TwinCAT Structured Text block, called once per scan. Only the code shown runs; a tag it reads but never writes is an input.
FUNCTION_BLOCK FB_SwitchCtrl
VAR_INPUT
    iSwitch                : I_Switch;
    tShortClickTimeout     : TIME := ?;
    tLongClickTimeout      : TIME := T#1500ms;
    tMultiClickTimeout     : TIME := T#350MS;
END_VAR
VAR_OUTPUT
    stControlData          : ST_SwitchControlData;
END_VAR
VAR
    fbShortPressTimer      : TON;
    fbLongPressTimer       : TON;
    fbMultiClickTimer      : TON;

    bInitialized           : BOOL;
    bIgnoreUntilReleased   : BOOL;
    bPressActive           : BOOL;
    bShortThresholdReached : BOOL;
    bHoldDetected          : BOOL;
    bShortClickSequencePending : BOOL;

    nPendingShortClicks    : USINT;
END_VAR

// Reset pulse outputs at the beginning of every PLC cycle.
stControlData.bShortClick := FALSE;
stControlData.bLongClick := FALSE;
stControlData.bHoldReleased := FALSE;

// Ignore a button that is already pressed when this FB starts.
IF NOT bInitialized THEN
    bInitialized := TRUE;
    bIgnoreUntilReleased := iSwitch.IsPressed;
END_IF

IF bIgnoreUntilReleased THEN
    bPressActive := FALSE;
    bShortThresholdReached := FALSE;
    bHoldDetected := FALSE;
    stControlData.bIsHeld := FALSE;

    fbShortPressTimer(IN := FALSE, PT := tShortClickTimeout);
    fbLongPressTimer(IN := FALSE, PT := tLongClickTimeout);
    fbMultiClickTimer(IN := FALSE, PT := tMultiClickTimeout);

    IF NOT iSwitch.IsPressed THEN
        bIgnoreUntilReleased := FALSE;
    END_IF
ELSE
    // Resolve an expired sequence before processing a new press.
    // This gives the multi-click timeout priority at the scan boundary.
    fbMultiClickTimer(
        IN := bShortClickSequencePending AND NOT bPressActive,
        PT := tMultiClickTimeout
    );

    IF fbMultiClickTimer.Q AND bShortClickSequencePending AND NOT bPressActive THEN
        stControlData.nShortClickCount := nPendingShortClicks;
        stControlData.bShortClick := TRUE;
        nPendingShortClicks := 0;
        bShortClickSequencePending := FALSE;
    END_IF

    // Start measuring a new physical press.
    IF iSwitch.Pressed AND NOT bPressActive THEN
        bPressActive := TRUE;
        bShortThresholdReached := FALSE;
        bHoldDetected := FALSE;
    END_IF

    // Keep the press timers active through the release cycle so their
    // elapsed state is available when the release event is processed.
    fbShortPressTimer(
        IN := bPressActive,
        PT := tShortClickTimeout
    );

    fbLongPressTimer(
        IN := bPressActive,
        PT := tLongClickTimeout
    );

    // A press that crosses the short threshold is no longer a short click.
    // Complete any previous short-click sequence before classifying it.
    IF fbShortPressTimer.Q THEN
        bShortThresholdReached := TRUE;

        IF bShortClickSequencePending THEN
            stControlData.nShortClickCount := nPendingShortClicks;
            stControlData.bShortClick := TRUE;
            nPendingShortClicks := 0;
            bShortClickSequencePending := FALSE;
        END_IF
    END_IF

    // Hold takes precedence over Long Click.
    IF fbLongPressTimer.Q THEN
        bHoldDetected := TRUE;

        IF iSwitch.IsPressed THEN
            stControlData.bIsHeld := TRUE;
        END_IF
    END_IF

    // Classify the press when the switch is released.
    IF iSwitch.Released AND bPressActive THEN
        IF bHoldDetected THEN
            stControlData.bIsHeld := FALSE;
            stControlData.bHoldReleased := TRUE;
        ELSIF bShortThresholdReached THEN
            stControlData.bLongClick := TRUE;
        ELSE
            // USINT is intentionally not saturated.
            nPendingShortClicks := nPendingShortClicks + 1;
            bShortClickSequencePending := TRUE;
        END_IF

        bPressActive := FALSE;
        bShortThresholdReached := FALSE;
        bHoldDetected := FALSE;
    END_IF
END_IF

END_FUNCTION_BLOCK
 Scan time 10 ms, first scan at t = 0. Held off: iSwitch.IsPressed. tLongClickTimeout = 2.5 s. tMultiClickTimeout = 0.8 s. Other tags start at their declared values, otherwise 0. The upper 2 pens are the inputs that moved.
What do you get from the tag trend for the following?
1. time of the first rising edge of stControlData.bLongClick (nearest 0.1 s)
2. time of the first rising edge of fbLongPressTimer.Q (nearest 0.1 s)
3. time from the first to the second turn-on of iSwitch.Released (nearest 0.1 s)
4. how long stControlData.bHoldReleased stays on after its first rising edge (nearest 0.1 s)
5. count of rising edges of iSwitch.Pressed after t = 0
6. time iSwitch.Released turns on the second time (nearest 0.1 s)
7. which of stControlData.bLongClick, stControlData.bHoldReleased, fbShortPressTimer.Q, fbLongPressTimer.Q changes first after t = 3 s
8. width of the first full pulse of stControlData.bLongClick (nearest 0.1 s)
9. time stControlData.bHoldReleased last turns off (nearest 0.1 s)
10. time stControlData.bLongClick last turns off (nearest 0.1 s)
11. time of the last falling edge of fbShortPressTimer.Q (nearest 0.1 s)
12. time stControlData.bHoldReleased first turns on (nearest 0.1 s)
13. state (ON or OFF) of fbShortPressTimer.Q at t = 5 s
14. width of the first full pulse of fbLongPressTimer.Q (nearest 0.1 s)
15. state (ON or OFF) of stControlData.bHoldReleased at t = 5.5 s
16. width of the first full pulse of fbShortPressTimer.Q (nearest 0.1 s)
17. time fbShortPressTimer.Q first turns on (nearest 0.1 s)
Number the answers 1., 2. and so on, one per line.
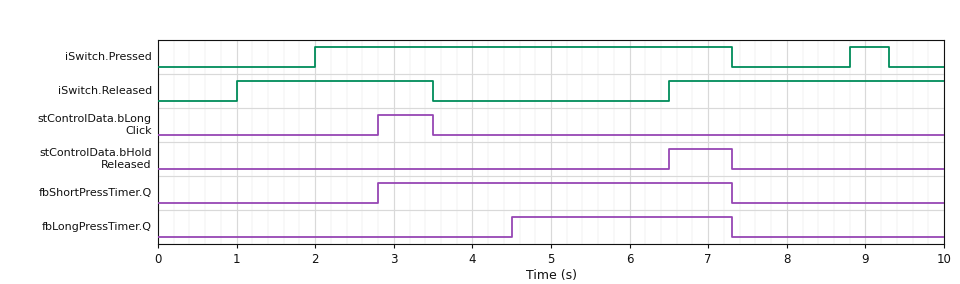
1. 2.8 s
2. 4.5 s
3. 5.5 s
4. 0.8 s
5. 2
6. 6.5 s
7. stControlData.bLongClick
8. 0.7 s
9. 7.3 s
10. 3.5 s
11. 7.3 s
12. 6.5 s
13. ON
14. 2.8 s
15. OFF
16. 4.5 s
17. 2.8 s
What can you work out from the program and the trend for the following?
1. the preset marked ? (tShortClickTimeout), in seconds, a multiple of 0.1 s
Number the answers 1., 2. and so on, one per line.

1. 0.8 s
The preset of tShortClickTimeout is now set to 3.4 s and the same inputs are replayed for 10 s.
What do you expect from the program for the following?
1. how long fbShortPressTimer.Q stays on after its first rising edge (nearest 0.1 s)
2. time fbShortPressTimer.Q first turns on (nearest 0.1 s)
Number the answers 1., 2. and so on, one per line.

1. 1.9 s
2. 5.4 s
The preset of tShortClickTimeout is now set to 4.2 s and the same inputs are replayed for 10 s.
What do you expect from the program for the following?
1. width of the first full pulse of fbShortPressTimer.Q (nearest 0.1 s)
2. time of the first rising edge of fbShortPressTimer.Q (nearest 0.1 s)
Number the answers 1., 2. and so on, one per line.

1. 1.1 s
2. 6.2 s
